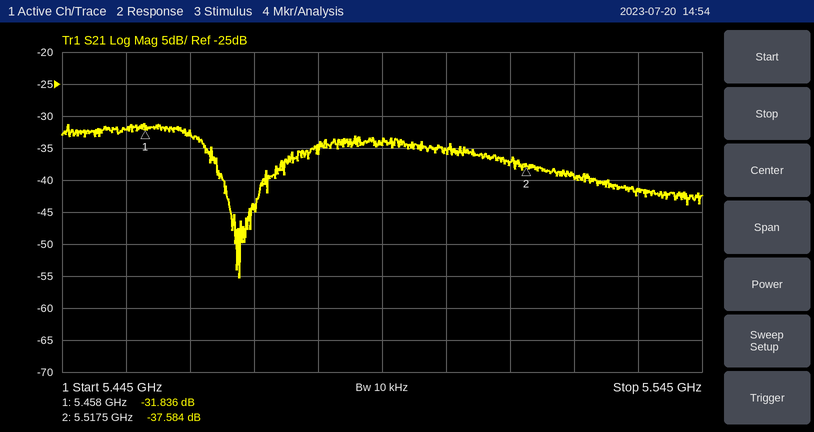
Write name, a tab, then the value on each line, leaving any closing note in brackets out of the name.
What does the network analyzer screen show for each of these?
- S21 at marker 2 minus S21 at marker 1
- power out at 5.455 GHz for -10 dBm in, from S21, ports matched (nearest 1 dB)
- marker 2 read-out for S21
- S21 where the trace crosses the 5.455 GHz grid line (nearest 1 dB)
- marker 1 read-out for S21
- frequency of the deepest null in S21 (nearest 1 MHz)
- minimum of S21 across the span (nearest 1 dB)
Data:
S21 at marker 2 minus S21 at marker 1	-5.748 dB
power out at 5.455 GHz for -10 dBm in, from S21, ports matched	-42 dBm
marker 2 read-out for S21	-37.584 dB
S21 where the trace crosses the 5.455 GHz grid line	-32 dB
marker 1 read-out for S21	-31.836 dB
frequency of the deepest null in S21	5.473 GHz
minimum of S21 across the span	-55 dB
